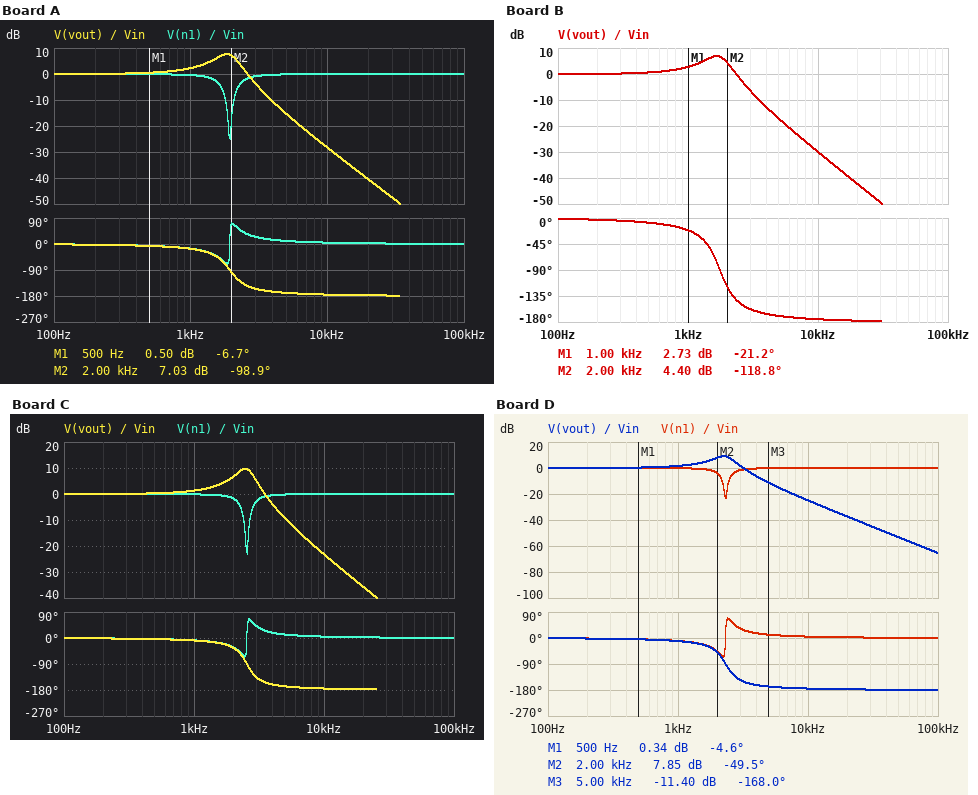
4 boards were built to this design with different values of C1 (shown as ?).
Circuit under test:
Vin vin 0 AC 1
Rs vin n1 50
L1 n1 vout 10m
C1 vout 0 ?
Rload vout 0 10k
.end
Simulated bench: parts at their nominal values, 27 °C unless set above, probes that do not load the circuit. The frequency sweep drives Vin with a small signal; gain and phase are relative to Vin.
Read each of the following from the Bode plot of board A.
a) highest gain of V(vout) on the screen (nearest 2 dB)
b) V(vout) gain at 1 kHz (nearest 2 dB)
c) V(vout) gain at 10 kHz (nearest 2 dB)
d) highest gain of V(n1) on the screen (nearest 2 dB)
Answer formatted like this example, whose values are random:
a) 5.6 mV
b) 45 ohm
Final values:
a) 8 dB
b) 2 dB
c) -28 dB
d) 0 dB
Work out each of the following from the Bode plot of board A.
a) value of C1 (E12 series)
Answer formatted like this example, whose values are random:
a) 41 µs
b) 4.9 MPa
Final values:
a) 680 nF
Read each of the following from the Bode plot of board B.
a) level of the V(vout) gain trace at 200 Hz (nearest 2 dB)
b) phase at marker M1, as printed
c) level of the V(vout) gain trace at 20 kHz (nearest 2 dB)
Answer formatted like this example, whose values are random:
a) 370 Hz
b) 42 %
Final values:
a) 0 dB
b) -21.2 deg
c) -42 dB
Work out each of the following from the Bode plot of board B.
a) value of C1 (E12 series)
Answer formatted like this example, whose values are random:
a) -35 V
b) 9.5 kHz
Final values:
a) 820 nF
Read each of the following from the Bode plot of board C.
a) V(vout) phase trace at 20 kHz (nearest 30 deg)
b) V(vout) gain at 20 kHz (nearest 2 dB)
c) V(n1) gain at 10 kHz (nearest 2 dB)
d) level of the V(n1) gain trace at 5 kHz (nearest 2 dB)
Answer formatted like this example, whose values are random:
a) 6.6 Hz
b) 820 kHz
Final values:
a) -180 deg
b) -36 dB
c) 0 dB
d) 0 dB
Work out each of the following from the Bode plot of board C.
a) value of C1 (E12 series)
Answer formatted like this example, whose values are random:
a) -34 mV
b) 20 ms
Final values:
a) 390 nF
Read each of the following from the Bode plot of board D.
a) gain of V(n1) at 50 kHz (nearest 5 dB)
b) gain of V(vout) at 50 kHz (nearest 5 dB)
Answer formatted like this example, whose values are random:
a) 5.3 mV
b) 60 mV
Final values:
a) 0 dB
b) -55 dB
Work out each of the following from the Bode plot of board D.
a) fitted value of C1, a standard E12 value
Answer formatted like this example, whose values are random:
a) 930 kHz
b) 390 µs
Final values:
a) 470 nF
